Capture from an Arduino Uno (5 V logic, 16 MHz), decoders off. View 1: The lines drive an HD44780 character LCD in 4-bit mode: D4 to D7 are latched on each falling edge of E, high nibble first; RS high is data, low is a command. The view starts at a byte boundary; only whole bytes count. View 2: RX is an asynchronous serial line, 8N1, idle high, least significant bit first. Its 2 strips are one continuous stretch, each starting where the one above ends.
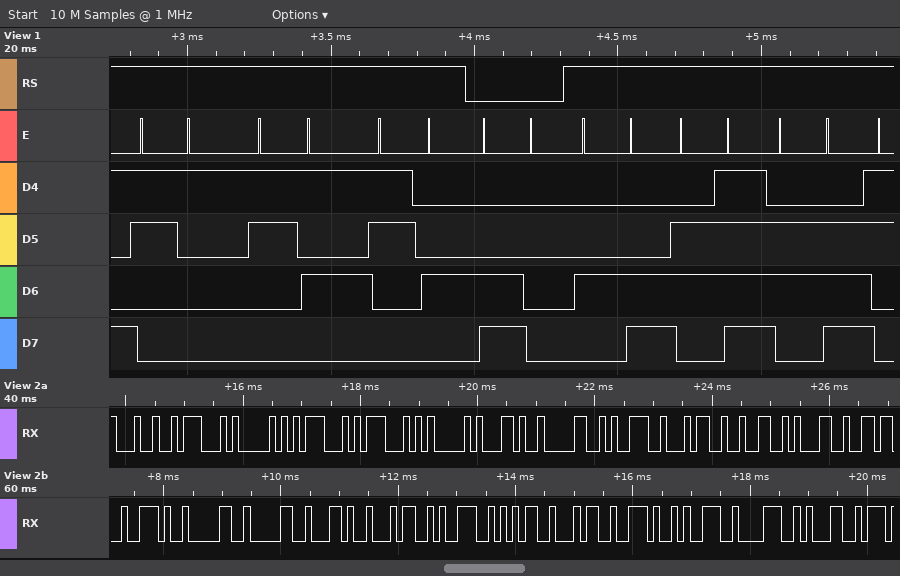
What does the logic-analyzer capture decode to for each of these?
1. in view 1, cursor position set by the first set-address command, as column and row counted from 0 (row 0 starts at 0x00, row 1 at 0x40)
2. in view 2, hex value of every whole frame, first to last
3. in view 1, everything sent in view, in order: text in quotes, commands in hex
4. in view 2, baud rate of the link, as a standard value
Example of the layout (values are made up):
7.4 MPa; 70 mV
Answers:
column 0, row 1; 24 47 50 47 47 41 2C 30 39 34 32 31 36 2E 30 30 2C 34 39 35 34 2E 39 38 31; "154" 0xC0 "Lon"; 9600 baud
